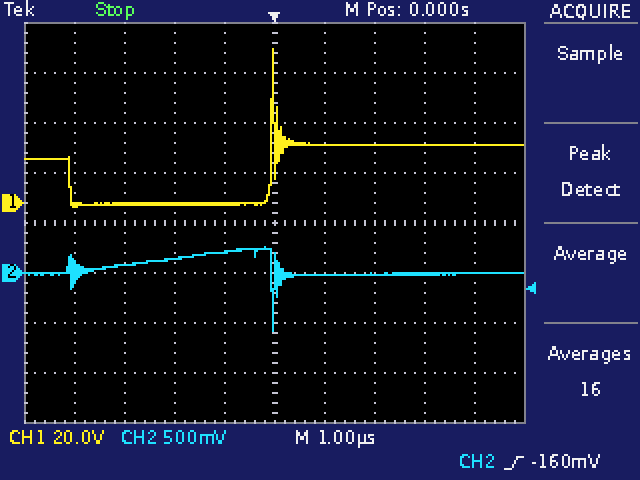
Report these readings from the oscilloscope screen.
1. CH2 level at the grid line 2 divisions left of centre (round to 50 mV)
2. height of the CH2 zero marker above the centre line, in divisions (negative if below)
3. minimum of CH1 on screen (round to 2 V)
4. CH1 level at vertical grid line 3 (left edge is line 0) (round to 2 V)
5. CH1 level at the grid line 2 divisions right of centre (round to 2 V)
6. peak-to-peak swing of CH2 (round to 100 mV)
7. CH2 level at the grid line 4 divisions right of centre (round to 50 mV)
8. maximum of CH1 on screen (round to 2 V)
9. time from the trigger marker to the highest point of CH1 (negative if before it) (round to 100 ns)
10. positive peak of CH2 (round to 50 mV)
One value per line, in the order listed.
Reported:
150 mV
-1.0 div
-2 V
0 V
24 V
800 mV
0 mV
62 V
0.0 µs
250 mV
